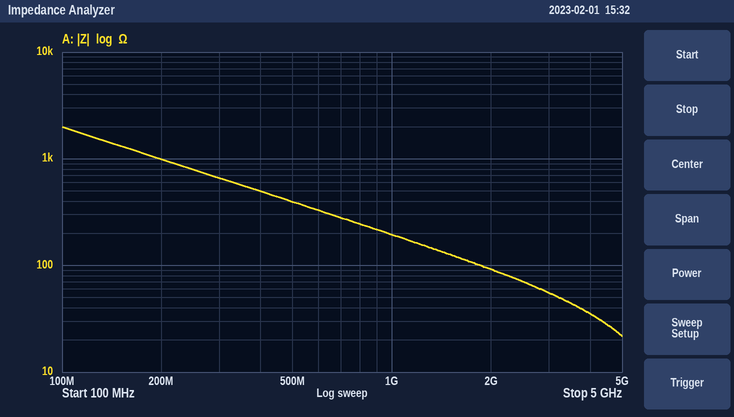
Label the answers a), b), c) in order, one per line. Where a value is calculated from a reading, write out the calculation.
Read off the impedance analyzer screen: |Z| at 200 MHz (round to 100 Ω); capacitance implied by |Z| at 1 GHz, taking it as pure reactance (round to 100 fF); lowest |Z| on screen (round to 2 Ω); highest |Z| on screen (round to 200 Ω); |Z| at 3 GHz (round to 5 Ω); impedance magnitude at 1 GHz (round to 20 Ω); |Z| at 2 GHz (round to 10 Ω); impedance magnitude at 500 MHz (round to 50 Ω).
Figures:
a) 1.0 kΩ
b) C = 1/(2π × 1 GHz × 200 Ω) ≈ 796 fF, so 800 fF to the nearest 100 fF
c) 22 Ω
d) 2.0 kΩ
e) 55 Ω
f) 200 Ω
g) 90 Ω
h) 400 Ω
